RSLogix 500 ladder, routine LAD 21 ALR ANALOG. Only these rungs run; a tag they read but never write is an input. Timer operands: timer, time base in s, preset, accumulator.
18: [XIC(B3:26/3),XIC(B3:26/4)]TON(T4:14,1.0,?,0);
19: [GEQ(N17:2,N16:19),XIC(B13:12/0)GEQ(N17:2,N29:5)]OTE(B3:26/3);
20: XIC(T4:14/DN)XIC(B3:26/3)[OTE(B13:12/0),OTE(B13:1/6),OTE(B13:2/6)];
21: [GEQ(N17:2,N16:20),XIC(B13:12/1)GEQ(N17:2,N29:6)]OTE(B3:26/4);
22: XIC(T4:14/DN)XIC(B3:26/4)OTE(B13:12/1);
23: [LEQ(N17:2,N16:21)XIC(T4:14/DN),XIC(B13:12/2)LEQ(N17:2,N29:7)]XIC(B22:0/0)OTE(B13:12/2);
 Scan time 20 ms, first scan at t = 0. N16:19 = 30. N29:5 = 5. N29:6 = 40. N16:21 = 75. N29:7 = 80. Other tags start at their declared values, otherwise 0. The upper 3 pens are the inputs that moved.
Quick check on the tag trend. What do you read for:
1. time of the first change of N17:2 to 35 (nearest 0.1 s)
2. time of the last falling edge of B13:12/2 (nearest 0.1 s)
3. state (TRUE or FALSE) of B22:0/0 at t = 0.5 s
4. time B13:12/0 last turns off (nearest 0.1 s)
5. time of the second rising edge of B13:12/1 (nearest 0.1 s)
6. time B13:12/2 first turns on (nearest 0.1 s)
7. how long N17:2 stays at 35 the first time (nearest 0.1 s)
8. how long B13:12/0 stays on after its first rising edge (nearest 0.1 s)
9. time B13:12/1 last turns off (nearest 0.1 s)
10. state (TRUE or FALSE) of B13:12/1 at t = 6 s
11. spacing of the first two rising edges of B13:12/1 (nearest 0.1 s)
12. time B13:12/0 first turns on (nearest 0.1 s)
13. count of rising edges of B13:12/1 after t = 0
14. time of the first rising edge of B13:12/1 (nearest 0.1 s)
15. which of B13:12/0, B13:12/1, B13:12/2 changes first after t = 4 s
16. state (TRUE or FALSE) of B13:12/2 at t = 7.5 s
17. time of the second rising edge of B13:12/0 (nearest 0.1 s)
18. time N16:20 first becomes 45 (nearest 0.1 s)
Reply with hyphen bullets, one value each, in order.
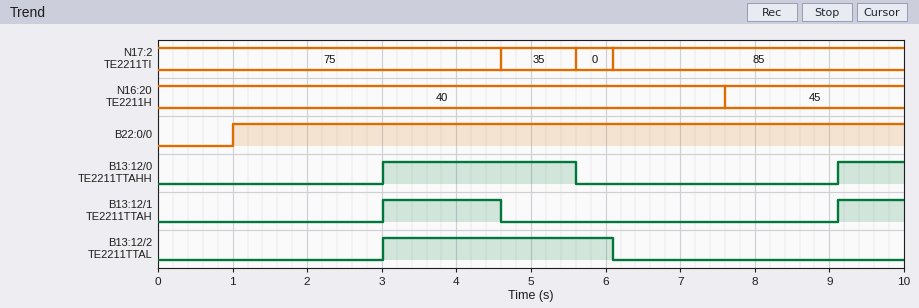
- 4.6 s
- 6.1 s
- FALSE
- 5.6 s
- 9.1 s
- 3.0 s
- 1.0 s
- 2.6 s
- 4.6 s
- FALSE
- 6.1 s
- 3.0 s
- 2
- 3.0 s
- B13:12/1
- FALSE
- 9.1 s
- 7.6 s
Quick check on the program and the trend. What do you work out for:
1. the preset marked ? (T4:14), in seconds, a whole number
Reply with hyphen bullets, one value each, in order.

- 3 s
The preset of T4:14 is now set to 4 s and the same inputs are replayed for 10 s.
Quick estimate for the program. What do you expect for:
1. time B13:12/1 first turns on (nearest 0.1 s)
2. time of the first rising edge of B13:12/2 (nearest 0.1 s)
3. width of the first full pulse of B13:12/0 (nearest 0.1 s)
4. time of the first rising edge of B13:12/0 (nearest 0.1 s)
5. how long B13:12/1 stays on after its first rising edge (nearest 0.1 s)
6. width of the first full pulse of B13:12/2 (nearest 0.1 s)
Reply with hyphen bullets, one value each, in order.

- 4.0 s
- 4.0 s
- 1.6 s
- 4.0 s
- 0.6 s
- 2.1 s
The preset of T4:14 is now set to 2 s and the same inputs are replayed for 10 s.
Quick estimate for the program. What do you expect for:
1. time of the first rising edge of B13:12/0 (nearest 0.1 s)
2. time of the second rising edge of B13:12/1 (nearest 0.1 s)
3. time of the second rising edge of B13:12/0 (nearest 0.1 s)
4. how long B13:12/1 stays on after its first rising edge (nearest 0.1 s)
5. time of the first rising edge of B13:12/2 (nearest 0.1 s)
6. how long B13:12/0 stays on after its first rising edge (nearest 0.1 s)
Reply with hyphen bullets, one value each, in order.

- 2.0 s
- 8.1 s
- 8.1 s
- 2.6 s
- 2.0 s
- 3.6 s
